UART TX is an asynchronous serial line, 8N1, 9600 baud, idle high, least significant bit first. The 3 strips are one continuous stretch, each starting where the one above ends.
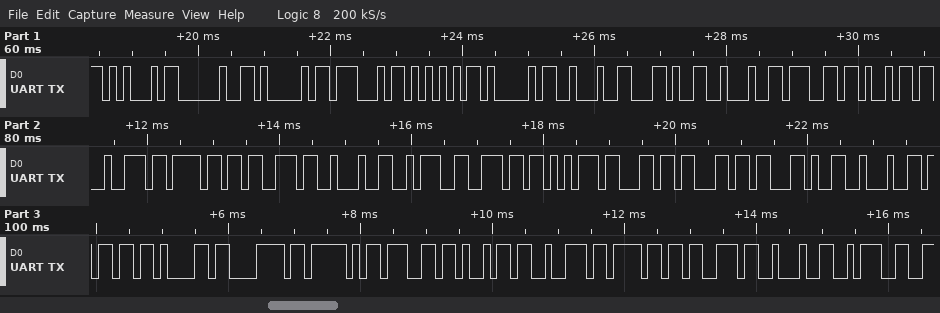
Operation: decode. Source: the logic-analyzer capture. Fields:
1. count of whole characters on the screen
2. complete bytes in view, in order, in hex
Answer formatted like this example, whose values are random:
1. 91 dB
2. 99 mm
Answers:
1. 33
2. 45 20 41 47 55 41 22 2C 22 67 69 72 6F 73 22 3A 6E 75 6C 6C 2C 22 6D 61 78 5F 67 69 72 6F 73 22 3A
